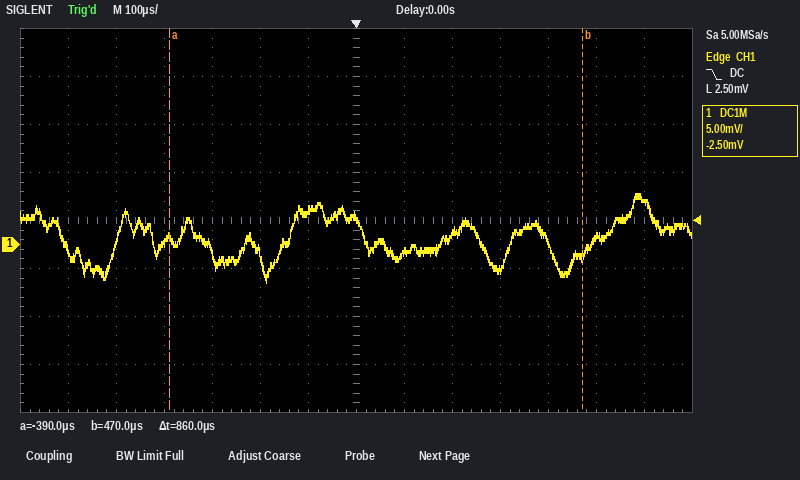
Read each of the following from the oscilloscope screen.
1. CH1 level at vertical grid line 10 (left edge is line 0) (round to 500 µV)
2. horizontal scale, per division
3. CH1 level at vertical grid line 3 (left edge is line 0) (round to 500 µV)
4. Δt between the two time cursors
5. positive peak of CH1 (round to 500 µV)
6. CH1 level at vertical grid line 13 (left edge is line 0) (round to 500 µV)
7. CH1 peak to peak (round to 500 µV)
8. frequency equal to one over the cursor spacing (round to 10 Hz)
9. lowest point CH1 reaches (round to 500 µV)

-2.5 mV
100 µs
0.0 mV
860 µs
5.5 mV
4.5 mV
9.5 mV
1.16 kHz
-4.0 mV
